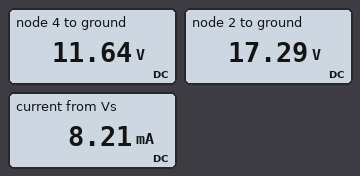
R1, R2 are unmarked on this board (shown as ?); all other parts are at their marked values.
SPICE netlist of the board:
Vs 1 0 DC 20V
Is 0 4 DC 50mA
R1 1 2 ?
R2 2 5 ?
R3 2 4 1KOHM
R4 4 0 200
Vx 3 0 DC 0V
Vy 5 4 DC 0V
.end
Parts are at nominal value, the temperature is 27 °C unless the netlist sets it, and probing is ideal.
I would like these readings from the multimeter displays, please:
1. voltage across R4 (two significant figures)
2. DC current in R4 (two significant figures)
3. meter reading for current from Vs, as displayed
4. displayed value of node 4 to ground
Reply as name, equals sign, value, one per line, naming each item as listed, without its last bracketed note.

voltage across R4 = 12 V
DC current in R4 = 58 mA
meter reading for current from Vs, as displayed = 8.21 mA
displayed value of node 4 to ground = 11.64 V
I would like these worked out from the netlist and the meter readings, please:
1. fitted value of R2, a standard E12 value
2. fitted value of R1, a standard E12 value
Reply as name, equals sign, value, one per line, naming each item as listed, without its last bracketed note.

fitted value of R2, a standard E12 value = 2.2 kΩ
fitted value of R1, a standard E12 value = 330 Ω
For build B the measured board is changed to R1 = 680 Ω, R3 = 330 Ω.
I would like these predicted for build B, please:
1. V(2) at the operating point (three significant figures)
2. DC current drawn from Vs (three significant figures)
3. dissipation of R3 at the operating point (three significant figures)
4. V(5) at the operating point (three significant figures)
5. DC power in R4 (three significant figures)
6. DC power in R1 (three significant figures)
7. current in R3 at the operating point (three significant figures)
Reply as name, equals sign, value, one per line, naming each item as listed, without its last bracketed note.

V(2) at the operating point = 14.2 V
DC current drawn from Vs = 8.57 mA
dissipation of R3 at the operating point = 18.3 mW
V(5) at the operating point = 11.7 V
DC power in R4 = 686 mW
DC power in R1 = 49.9 mW
current in R3 at the operating point = 7.45 mA
